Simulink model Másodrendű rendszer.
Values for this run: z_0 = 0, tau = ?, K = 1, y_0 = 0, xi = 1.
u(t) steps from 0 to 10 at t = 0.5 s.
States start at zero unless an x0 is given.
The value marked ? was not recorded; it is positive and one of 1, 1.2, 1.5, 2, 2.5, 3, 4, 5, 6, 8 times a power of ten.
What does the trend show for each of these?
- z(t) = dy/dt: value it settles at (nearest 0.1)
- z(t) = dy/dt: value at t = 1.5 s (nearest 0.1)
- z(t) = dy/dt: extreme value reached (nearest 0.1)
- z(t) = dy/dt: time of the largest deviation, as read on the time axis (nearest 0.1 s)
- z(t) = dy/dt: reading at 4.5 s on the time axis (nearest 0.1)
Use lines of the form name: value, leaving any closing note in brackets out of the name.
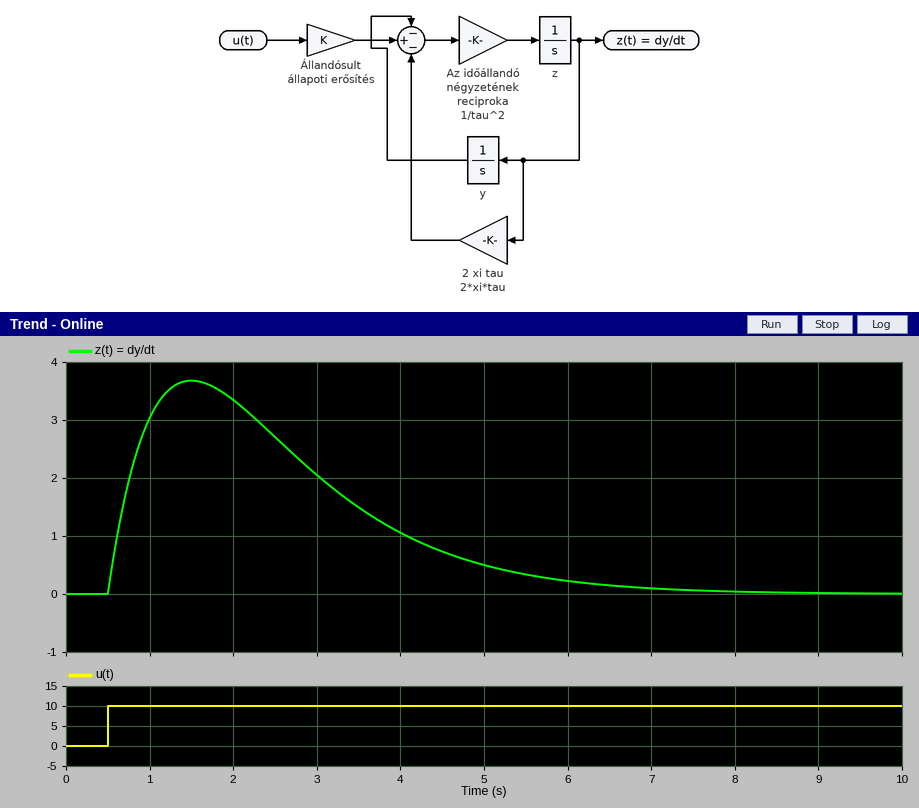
z(t) = dy/dt: value it settles at: 0.0
z(t) = dy/dt: value at t = 1.5 s: 3.7
z(t) = dy/dt: extreme value reached: 3.7
z(t) = dy/dt: time of the largest deviation, as read on the time axis: 1.5 s
z(t) = dy/dt: reading at 4.5 s on the time axis: 0.7
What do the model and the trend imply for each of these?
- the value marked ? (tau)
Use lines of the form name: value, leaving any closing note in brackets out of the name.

the value marked ?: 1
